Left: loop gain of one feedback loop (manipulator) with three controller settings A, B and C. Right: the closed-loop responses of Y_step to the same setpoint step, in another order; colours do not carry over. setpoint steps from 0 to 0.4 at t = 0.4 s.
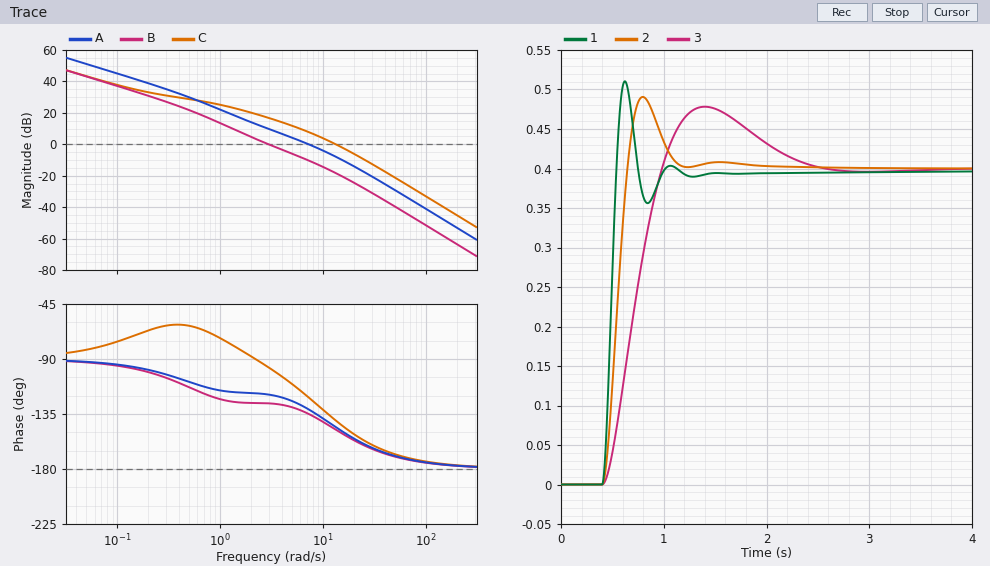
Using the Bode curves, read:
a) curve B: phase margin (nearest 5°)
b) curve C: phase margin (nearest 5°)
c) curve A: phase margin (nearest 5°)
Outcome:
55°
40°
50°
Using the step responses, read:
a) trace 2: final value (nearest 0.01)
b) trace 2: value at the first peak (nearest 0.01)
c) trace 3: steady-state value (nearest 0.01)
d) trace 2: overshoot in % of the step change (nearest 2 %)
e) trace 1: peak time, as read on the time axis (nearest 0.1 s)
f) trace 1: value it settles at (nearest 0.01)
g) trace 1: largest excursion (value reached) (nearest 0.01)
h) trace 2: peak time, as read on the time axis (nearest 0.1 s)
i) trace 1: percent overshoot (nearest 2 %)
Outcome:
0.40
0.49
0.40
22 %
0.6 s
0.40
0.51
0.8 s
28 %
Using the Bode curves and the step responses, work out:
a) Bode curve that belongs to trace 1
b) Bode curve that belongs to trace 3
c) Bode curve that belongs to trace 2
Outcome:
C
B
A
